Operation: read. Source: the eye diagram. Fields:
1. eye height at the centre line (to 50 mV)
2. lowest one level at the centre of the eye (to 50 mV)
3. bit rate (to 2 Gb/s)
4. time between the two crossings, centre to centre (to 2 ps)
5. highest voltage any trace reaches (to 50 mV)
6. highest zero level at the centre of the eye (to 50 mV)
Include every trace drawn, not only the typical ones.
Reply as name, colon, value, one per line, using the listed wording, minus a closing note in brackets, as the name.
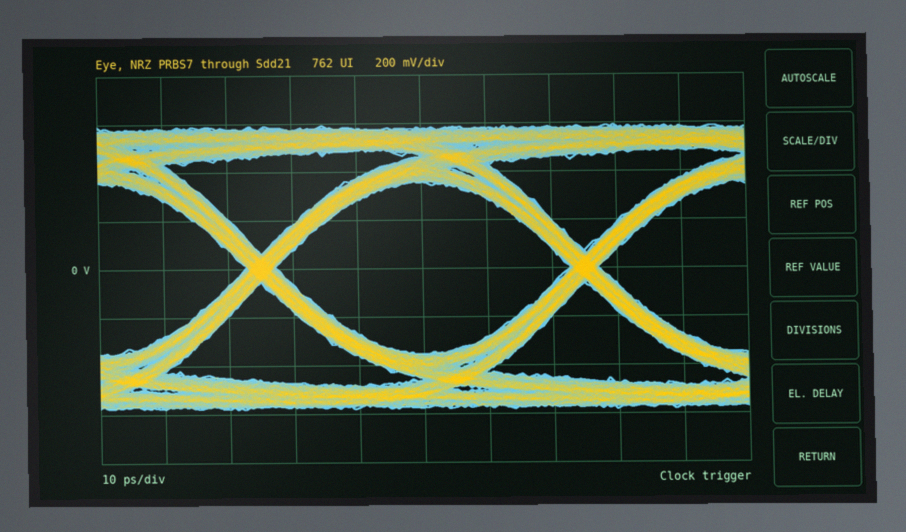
eye height at the centre line: 700 mV
lowest one level at the centre of the eye: 350 mV
bit rate: 20 Gb/s
time between the two crossings, centre to centre: 50 ps
highest voltage any trace reaches: 600 mV
highest zero level at the centre of the eye: -350 mV
